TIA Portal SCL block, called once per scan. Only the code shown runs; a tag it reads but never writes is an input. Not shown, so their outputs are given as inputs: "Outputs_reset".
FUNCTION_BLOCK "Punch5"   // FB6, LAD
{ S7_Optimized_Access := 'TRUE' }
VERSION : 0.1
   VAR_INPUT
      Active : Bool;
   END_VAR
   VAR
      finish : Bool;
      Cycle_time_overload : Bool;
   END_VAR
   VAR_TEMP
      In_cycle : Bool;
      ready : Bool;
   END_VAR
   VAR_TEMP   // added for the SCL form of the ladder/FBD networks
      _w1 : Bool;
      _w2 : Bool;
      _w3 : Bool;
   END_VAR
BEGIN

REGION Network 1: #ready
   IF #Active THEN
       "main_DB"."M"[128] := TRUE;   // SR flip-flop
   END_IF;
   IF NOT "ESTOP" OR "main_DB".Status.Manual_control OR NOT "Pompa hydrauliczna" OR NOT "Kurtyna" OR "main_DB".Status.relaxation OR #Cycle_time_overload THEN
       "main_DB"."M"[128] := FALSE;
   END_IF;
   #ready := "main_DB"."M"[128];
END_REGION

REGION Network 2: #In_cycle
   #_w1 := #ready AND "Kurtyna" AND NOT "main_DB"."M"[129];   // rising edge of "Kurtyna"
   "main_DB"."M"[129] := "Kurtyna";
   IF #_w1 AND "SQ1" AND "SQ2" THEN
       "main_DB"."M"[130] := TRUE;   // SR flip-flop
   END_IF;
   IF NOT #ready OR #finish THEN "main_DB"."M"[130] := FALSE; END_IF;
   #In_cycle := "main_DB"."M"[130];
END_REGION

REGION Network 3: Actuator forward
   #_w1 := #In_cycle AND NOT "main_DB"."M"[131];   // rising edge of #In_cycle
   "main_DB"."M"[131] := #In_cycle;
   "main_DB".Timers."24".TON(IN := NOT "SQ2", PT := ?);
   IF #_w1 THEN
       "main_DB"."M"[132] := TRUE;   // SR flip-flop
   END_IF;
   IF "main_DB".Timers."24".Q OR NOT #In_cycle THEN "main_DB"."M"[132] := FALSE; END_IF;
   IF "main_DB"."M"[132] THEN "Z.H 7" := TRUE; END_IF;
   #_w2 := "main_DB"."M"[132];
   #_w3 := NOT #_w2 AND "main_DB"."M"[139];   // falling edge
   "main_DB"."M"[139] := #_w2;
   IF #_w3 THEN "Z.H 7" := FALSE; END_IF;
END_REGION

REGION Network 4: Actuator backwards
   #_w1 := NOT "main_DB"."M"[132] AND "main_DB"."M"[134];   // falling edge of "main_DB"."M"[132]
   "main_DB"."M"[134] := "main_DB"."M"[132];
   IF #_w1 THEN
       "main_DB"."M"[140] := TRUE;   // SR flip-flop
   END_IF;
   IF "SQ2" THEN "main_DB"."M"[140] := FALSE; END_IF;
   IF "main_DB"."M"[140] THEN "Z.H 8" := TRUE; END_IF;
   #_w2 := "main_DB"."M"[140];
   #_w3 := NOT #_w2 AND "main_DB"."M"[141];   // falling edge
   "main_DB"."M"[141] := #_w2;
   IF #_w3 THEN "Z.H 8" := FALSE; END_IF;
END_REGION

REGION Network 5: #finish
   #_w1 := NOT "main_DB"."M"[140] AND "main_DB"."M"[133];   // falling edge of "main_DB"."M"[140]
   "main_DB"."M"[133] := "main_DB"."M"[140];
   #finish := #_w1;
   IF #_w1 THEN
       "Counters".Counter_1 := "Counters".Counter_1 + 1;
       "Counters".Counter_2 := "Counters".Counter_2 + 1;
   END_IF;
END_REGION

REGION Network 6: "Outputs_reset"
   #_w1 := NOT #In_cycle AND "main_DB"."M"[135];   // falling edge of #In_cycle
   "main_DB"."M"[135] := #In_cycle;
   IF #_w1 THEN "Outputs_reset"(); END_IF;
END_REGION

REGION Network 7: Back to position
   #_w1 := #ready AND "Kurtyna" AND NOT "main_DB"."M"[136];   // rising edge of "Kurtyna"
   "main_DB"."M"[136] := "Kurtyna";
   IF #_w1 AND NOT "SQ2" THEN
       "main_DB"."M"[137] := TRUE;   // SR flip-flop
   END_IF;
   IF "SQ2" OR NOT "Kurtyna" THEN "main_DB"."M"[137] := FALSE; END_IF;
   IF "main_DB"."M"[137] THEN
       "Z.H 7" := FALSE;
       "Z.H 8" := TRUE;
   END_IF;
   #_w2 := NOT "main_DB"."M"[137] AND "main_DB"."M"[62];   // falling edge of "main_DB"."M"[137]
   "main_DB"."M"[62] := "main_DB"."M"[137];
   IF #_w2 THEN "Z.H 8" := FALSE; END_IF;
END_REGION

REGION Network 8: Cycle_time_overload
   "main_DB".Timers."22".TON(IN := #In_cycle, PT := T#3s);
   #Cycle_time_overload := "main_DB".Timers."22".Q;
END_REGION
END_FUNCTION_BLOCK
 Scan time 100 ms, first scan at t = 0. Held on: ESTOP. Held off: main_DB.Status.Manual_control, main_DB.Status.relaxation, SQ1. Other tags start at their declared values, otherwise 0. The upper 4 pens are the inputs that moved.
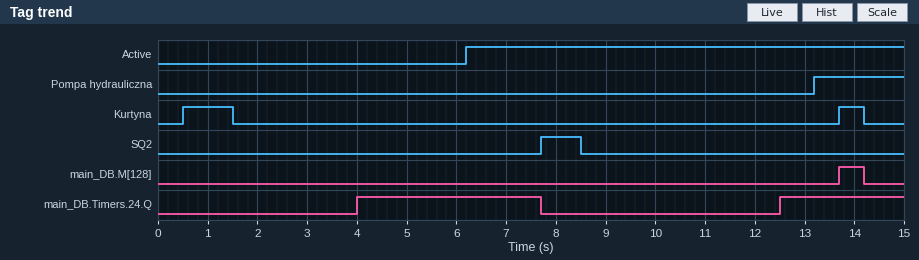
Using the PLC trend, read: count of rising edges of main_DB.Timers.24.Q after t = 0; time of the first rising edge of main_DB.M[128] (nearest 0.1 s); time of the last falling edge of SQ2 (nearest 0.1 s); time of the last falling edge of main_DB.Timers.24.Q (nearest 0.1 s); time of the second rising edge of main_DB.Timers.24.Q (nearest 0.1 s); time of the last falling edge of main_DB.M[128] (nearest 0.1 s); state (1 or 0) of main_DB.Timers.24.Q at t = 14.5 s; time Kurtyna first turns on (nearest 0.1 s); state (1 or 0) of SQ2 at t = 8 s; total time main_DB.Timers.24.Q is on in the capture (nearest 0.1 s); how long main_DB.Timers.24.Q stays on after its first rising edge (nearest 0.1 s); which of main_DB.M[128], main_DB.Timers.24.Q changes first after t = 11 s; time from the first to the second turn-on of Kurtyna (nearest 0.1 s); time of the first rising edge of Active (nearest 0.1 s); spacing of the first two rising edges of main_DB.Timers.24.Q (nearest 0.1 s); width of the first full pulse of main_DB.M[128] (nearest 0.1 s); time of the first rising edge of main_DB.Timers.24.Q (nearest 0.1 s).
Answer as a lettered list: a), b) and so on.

a) 2
b) 13.7 s
c) 8.5 s
d) 7.7 s
e) 12.5 s
f) 14.2 s
g) 1
h) 0.5 s
i) 1
j) 6.2 s
k) 3.7 s
l) main_DB.Timers.24.Q
m) 13.2 s
n) 6.2 s
o) 8.5 s
p) 0.5 s
q) 4.0 s
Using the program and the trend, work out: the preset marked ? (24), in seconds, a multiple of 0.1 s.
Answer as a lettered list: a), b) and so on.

a) 4.0 s
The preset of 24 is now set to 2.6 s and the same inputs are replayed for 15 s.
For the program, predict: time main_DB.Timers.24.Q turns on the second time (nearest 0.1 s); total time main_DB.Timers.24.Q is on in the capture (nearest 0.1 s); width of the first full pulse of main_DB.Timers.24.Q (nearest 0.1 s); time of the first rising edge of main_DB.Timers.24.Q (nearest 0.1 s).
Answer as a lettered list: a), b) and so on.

a) 11.1 s
b) 9.0 s
c) 5.1 s
d) 2.6 s
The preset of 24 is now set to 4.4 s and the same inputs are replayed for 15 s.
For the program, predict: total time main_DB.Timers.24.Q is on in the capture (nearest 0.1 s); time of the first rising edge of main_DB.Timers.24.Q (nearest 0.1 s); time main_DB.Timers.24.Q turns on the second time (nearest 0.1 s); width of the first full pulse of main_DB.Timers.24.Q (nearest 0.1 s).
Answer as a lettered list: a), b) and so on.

a) 5.4 s
b) 4.4 s
c) 12.9 s
d) 3.3 s
